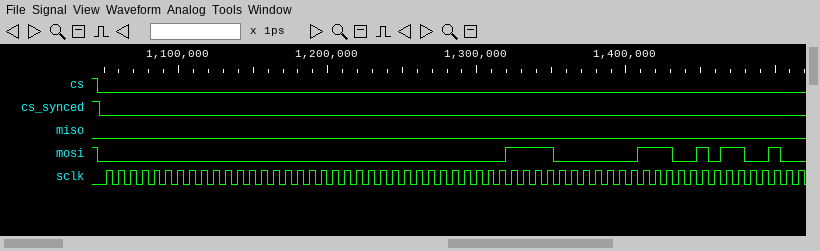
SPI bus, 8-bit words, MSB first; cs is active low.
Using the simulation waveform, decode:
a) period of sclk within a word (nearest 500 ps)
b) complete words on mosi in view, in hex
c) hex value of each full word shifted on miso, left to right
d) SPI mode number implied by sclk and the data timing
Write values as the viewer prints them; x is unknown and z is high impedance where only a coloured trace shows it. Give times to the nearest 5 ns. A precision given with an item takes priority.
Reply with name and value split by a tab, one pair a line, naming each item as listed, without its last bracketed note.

period of sclk within a word	8000 ps
complete words on mosi in view, in hex	00, 00, 00, 00, 3C, 07, 2C
hex value of each full word shifted on miso, left to right	00, 00, 00, 00, 00, 00, 00
SPI mode number implied by sclk and the data timing	0
